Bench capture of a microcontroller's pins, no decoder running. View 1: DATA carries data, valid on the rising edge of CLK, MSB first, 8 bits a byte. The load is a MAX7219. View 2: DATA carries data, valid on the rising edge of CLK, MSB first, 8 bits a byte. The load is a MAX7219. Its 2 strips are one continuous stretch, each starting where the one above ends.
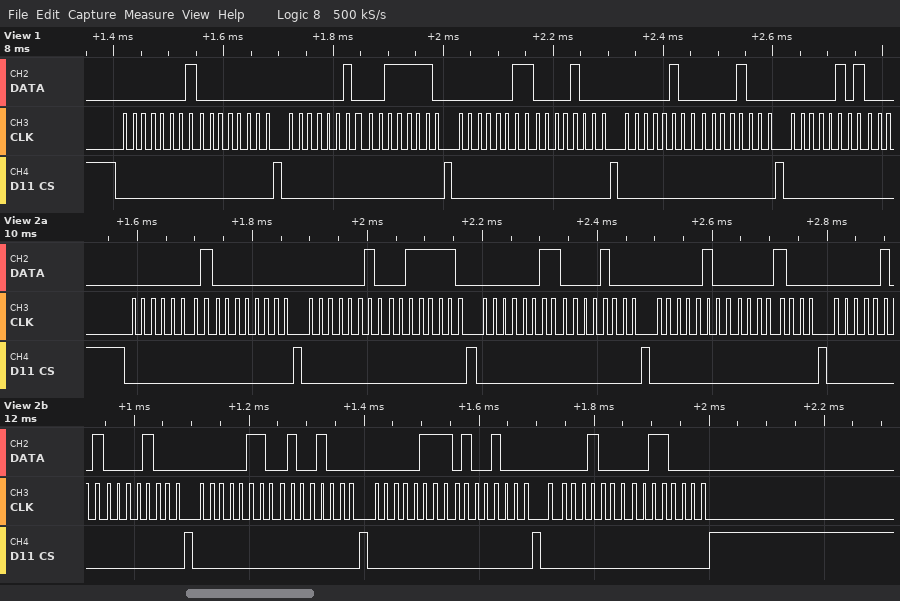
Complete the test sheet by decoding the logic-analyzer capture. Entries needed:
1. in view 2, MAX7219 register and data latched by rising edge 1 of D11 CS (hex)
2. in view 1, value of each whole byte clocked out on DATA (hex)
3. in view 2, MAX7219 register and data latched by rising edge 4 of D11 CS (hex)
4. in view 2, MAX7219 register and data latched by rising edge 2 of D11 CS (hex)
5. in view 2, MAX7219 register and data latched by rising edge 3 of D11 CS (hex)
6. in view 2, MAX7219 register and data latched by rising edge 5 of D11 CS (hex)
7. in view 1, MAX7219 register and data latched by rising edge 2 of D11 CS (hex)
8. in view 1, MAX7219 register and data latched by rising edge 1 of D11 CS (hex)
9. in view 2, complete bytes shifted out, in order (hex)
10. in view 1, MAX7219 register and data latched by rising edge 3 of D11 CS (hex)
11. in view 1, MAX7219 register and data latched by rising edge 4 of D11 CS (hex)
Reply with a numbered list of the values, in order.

1. register 0x1, data 0x00
2. 0x01 0x00 0x02 0x3E 0x03 0x08 0x04 0x08 0x05
3. register 0x4, data 0x08
4. register 0x2, data 0x3E
5. register 0x3, data 0x08
6. register 0x5, data 0x08
7. register 0x2, data 0x3E
8. register 0x1, data 0x00
9. 0x01 0x00 0x02 0x3E 0x03 0x08 0x04 0x08 0x05 0x08 0x06 0x48 0x07 0x48 0x08 0x30
10. register 0x3, data 0x08
11. register 0x4, data 0x08
